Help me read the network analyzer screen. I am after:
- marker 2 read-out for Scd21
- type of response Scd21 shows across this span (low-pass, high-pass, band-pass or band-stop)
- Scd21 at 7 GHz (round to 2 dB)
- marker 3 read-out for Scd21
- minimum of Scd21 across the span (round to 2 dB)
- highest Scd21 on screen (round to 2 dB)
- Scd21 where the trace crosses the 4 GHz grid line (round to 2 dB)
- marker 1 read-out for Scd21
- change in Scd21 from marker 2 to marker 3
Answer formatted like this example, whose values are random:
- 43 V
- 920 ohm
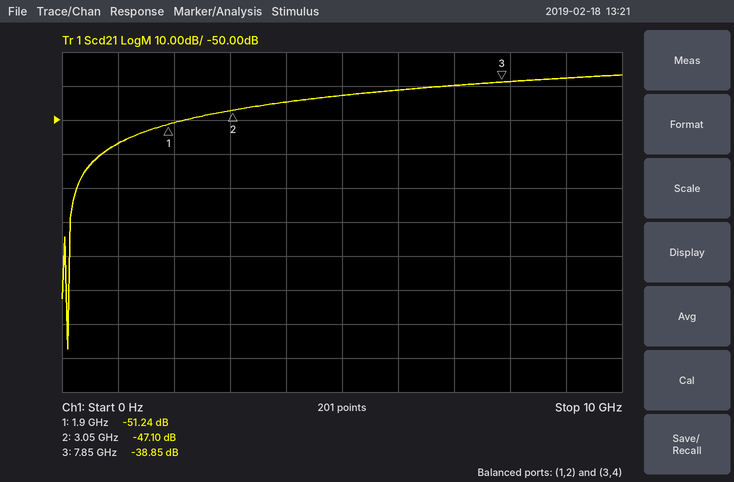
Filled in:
- -47.10 dB
- high-pass
- -40 dB
- -38.85 dB
- -118 dB
- -36 dB
- -44 dB
- -51.24 dB
- 8.25 dB
